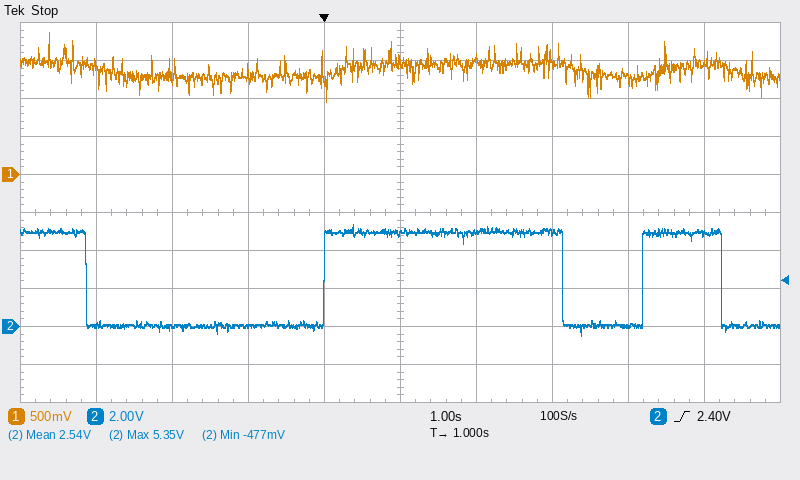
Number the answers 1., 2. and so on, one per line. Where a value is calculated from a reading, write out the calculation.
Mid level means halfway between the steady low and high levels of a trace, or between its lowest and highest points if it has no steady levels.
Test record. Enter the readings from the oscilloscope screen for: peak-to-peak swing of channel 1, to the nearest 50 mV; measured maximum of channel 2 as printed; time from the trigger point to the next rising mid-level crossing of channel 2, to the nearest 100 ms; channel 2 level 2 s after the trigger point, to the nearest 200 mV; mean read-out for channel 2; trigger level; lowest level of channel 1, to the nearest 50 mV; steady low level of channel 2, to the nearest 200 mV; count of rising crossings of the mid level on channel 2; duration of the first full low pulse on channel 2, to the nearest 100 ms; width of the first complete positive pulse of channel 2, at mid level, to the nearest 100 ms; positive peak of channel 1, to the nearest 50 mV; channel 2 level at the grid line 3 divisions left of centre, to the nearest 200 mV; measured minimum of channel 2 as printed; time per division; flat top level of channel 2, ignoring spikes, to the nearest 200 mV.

1. 1.85 V − (950 mV) = 900 mV
2. 5.35 V
3. 4.2 s
4. 5.0 V
5. 2.54 V
6. 2.40 V
7. 950 mV
8. 0.0 V
9. 2
10. 3.1 s
11. 3.1 s
12. 1.85 V
13. 0.0 V
14. -477 mV
15. 1 s
16. 5.0 V
